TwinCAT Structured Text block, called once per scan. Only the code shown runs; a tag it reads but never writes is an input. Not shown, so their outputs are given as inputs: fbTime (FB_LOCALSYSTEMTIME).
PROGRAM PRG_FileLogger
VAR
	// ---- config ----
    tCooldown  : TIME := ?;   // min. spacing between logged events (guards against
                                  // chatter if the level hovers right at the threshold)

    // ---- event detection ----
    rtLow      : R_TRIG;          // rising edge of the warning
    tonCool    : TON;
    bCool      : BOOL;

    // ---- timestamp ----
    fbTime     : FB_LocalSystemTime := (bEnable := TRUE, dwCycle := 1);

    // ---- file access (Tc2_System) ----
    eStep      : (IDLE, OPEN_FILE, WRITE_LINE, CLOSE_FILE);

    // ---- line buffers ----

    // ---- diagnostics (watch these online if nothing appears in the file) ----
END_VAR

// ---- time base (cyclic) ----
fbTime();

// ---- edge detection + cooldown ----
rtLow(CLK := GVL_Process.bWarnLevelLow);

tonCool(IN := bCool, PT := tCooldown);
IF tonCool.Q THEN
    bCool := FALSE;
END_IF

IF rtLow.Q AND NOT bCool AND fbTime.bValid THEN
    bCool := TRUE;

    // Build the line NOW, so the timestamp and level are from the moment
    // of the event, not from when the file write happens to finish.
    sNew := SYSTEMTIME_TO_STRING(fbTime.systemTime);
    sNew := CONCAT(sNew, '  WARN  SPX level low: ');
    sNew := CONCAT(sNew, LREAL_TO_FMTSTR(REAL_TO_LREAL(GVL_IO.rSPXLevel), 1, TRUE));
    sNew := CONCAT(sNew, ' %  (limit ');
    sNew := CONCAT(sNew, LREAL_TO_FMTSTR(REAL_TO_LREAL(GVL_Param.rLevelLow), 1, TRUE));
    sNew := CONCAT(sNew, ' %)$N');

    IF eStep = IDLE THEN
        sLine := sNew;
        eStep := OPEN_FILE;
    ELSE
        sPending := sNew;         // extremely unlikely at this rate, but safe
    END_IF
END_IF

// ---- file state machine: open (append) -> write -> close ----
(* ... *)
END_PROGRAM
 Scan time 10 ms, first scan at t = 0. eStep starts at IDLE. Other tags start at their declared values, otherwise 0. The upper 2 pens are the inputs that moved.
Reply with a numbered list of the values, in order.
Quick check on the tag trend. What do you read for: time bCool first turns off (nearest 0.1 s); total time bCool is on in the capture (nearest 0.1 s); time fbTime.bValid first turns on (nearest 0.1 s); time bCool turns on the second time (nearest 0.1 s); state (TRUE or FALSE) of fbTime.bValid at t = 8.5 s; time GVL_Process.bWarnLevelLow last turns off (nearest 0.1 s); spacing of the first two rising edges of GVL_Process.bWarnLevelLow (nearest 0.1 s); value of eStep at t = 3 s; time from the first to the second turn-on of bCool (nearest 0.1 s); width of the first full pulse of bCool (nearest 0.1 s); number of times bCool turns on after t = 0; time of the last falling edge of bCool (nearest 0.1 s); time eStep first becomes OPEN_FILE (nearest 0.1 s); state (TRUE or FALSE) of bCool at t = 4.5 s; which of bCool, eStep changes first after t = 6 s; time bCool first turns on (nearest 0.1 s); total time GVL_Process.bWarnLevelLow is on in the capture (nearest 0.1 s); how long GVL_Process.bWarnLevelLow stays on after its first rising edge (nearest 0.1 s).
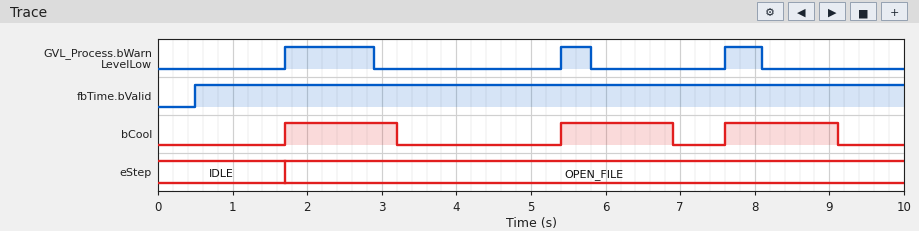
1. 3.2 s
2. 4.5 s
3. 0.5 s
4. 5.4 s
5. TRUE
6. 8.1 s
7. 3.7 s
8. OPEN_FILE
9. 3.7 s
10. 1.5 s
11. 3
12. 9.1 s
13. 1.7 s
14. FALSE
15. bCool
16. 1.7 s
17. 2.1 s
18. 1.2 s
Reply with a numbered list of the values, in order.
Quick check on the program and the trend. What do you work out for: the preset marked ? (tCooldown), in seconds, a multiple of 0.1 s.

1. 1.5 s
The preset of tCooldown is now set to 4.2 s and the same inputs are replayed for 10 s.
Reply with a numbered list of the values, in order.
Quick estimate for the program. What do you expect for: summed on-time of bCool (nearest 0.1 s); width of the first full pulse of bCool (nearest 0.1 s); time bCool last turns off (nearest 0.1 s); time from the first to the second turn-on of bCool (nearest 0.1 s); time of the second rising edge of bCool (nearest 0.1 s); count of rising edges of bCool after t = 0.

1. 6.6 s
2. 4.2 s
3. 5.9 s
4. 5.9 s
5. 7.6 s
6. 2
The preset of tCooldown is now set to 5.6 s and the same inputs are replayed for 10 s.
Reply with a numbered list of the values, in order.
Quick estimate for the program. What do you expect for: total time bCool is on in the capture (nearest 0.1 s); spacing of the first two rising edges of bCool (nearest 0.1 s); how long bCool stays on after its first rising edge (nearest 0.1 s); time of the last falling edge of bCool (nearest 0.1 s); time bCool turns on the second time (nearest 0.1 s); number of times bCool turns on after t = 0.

1. 8.0 s
2. 5.9 s
3. 5.6 s
4. 7.3 s
5. 7.6 s
6. 2
